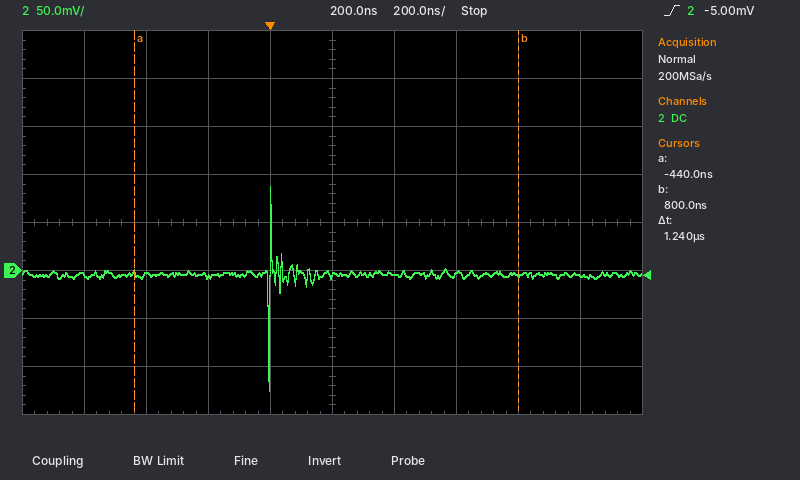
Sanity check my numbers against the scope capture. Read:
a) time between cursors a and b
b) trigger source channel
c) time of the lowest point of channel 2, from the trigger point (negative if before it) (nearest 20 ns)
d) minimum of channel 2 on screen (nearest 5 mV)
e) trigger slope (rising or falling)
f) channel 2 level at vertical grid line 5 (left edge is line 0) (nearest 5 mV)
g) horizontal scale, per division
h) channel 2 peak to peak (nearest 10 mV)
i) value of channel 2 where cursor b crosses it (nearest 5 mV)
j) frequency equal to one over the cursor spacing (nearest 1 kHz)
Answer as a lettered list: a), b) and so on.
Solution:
a) 1.24 µs
b) channel 2
c) 0 ns
d) -125 mV
e) rising
f) -5 mV
g) 200 ns
h) 210 mV
i) -5 mV
j) 806 kHz
